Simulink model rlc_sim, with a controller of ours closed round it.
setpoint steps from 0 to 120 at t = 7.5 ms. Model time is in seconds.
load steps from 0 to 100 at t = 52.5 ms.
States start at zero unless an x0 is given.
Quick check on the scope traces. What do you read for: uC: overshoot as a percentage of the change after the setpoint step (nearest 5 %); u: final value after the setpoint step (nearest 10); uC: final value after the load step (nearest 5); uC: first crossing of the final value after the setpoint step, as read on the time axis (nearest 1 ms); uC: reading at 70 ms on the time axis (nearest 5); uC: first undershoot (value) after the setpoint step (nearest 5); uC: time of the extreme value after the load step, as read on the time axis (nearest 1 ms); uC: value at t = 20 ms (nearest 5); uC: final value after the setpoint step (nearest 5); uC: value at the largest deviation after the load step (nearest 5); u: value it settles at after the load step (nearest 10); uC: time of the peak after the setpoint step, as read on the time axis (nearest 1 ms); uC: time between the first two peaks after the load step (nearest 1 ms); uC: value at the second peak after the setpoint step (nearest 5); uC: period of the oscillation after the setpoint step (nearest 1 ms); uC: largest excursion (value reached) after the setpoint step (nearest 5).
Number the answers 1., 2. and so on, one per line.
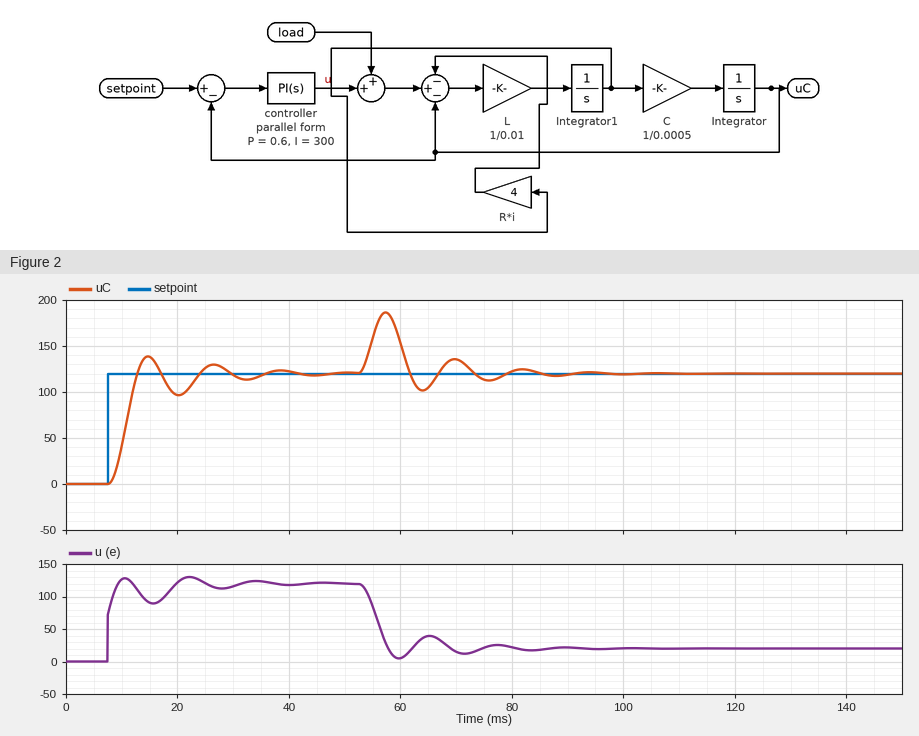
1. 15 %
2. 120
3. 120
4. 13 ms
5. 135
6. 95
7. 57 ms
8. 95
9. 120
10. 185
11. 20
12. 15 ms
13. 12 ms
14. 130
15. 12 ms
16. 140
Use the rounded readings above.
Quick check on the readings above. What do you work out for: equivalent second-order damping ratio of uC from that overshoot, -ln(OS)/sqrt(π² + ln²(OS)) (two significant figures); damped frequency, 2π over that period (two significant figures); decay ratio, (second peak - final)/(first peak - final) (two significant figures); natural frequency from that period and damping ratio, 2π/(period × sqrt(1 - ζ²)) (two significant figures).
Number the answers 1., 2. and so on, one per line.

1. 0.52
2. 0.52 rad/ms
3. 0.50
4. 0.61 rad/ms
